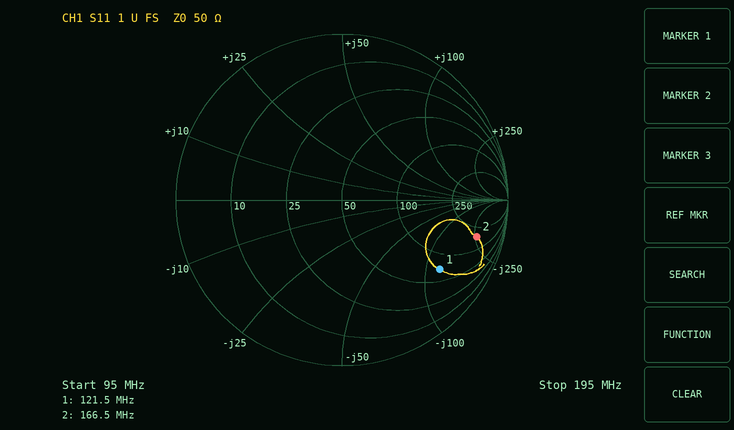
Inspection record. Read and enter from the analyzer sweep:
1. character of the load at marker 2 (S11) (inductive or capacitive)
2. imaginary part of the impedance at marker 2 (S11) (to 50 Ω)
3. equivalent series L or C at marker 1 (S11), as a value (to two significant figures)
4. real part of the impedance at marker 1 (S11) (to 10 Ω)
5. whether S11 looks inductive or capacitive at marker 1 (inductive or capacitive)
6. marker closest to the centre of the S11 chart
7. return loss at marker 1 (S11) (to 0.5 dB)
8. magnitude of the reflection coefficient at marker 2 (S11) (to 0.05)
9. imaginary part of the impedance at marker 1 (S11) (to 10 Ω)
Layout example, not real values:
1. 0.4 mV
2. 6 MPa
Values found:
1. capacitive
2. -250 Ω
3. 11 pF
4. 70 Ω
5. capacitive
6. marker 1
7. 3.0 dB
8. 0.85
9. -120 Ω
